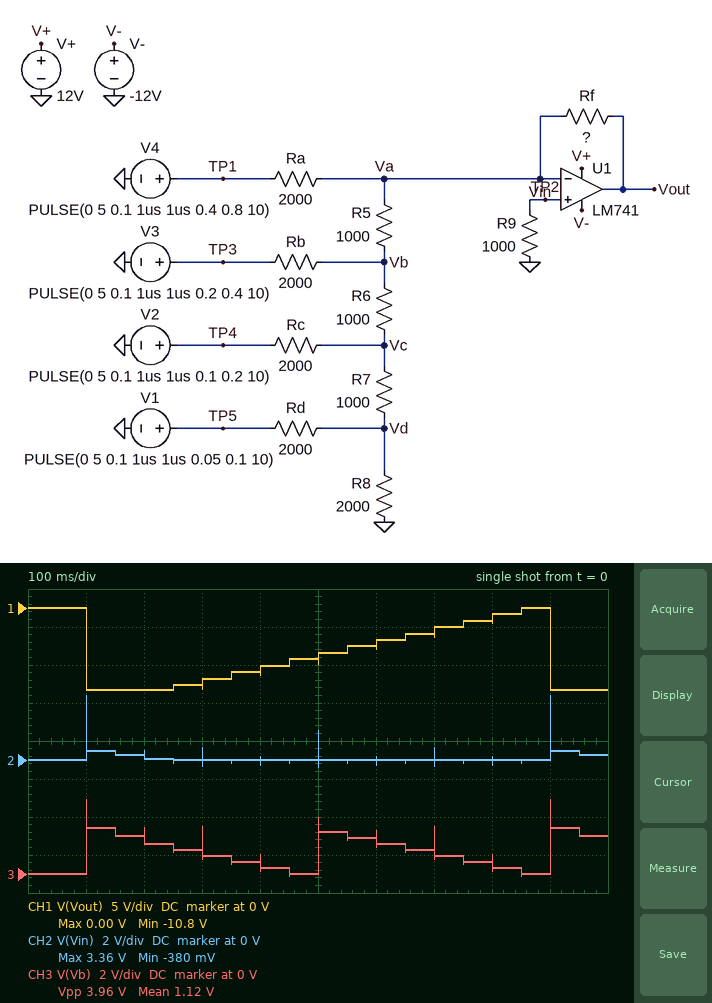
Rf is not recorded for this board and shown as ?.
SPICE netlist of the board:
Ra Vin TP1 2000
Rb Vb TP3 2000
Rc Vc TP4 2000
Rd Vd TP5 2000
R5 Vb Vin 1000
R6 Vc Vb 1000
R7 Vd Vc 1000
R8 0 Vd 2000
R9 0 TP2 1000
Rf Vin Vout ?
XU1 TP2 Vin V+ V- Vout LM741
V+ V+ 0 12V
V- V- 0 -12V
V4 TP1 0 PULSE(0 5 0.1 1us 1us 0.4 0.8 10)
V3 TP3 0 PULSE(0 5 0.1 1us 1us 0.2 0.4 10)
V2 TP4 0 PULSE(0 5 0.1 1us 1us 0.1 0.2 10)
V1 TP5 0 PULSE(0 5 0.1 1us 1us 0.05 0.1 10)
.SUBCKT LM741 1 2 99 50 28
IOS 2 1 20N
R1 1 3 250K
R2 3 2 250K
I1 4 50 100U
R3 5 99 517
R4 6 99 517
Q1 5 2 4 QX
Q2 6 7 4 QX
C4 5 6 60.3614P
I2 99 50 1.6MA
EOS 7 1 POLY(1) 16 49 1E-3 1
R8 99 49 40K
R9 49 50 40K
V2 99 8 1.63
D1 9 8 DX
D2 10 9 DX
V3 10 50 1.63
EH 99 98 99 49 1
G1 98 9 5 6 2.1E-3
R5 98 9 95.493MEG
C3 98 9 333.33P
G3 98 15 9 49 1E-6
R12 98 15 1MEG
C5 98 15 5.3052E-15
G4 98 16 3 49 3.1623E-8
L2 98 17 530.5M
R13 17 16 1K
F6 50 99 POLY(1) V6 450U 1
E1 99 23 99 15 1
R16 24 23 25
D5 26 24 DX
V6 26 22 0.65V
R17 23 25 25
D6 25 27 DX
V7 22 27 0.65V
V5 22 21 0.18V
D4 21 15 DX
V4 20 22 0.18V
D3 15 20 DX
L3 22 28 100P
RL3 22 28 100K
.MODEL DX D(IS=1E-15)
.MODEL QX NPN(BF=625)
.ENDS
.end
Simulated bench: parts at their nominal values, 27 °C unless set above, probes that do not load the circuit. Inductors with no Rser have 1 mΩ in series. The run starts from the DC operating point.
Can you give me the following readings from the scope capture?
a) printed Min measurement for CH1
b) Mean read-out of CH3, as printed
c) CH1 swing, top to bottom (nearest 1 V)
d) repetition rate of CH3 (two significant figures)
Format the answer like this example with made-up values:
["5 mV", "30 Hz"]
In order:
["-10.8 V", "1.12 V", "11 V", "2.5 Hz"]
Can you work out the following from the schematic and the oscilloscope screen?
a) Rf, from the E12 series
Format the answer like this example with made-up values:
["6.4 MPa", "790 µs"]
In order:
["2.7 kΩ"]
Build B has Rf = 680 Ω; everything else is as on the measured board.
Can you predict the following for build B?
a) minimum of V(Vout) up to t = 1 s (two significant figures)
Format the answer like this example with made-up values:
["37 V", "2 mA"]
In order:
["-3.2 V"]
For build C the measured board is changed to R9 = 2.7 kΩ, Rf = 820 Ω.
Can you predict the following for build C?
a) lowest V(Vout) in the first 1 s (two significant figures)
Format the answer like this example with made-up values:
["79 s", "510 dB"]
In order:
["-3.8 V"]
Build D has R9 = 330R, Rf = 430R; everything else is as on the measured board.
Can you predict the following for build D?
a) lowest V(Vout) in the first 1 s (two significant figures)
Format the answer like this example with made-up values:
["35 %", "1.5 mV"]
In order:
["-2.0 V"]
